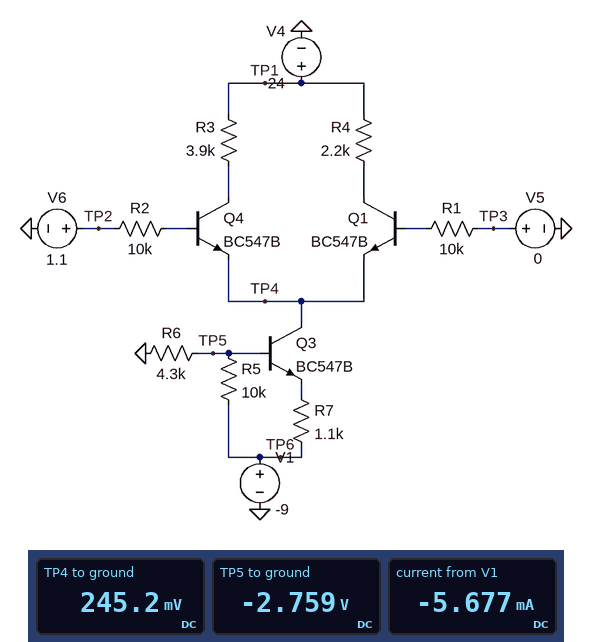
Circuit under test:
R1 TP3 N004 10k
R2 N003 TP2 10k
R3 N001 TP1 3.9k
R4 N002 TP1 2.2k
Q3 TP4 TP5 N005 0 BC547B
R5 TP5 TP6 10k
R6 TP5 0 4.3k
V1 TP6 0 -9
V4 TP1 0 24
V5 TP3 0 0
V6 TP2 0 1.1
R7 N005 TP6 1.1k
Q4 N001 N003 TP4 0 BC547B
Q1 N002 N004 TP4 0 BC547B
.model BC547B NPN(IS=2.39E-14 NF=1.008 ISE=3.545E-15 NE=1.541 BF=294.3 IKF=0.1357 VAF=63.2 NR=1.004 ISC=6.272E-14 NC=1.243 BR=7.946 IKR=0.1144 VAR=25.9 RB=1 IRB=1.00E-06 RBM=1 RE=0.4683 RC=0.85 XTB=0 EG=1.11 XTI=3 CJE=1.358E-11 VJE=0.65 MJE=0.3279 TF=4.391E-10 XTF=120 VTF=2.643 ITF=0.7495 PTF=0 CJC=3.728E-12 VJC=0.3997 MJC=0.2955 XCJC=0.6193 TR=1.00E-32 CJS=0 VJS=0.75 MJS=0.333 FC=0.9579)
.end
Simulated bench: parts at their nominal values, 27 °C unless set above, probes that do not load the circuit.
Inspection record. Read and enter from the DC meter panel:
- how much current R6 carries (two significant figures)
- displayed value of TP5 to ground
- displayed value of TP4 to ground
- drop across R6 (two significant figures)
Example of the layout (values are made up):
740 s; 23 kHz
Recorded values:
640 µA; -2.759 V; 245.2 mV; 2.8 V
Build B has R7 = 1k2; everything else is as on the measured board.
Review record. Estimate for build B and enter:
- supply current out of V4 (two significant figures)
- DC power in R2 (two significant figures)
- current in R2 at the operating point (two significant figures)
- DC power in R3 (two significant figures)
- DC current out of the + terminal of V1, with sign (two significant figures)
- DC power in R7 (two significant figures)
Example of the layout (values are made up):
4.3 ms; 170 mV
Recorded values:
4.6 mA; 2.4 µW; 15 µA; 83 mW; -5.3 mA; 26 mW
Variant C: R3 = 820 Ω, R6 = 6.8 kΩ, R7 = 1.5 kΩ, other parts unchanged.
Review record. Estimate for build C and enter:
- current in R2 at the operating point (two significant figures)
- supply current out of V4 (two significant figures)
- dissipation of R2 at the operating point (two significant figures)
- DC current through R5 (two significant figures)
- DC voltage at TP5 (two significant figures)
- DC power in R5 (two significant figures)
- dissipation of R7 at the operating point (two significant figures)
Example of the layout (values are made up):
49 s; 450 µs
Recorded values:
8.3 µA; 3.1 mA; 680 nW; 530 µA; -3.7 V; 2.8 mW; 14 mW
